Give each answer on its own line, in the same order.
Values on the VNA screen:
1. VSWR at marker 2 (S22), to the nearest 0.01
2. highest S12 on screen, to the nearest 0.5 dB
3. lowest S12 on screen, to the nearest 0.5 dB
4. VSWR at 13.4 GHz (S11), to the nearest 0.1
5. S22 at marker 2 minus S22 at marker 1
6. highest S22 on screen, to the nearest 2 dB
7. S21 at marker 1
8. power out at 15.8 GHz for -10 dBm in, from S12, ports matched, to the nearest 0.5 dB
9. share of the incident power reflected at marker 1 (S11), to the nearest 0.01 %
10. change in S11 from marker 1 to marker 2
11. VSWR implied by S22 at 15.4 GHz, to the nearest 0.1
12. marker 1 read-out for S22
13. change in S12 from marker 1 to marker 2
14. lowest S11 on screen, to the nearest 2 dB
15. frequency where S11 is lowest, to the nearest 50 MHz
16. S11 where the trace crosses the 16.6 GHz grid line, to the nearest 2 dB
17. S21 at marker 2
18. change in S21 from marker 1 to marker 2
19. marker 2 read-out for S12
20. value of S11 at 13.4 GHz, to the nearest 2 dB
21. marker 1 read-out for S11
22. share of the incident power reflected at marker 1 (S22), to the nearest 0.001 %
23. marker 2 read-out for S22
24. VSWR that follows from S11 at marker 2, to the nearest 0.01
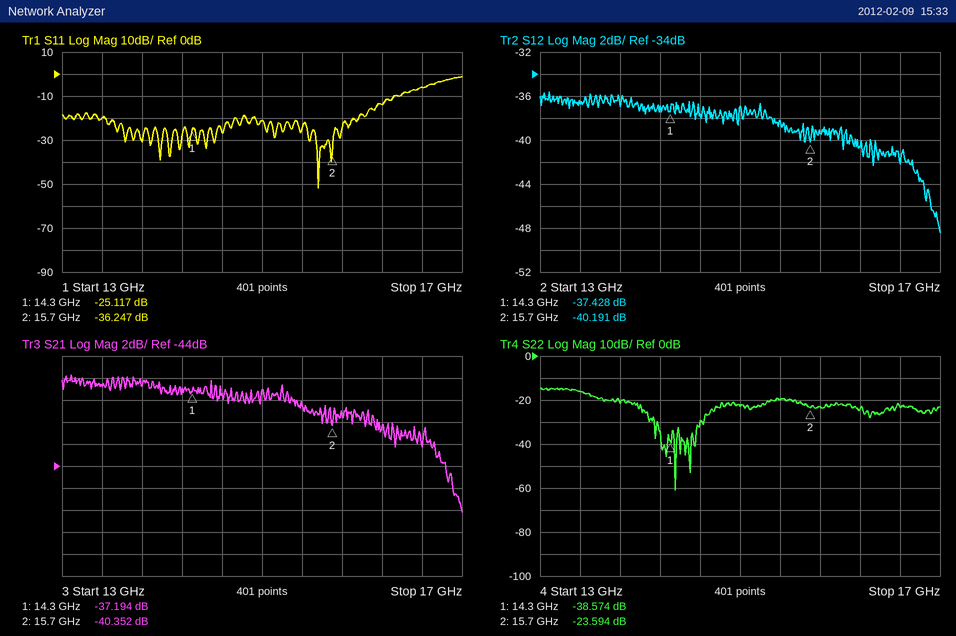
1.14
-35.5 dB
-48.5 dB
1.2
14.980 dB
-14 dB
-37.194 dB
-49.5 dBm
0.31 %
-11.130 dB
1.2
-38.574 dB
-2.763 dB
-52 dB
15.55 GHz
-6 dB
-40.352 dB
-3.158 dB
-40.191 dB
-20 dB
-25.117 dB
0.014 %
-23.594 dB
1.03
